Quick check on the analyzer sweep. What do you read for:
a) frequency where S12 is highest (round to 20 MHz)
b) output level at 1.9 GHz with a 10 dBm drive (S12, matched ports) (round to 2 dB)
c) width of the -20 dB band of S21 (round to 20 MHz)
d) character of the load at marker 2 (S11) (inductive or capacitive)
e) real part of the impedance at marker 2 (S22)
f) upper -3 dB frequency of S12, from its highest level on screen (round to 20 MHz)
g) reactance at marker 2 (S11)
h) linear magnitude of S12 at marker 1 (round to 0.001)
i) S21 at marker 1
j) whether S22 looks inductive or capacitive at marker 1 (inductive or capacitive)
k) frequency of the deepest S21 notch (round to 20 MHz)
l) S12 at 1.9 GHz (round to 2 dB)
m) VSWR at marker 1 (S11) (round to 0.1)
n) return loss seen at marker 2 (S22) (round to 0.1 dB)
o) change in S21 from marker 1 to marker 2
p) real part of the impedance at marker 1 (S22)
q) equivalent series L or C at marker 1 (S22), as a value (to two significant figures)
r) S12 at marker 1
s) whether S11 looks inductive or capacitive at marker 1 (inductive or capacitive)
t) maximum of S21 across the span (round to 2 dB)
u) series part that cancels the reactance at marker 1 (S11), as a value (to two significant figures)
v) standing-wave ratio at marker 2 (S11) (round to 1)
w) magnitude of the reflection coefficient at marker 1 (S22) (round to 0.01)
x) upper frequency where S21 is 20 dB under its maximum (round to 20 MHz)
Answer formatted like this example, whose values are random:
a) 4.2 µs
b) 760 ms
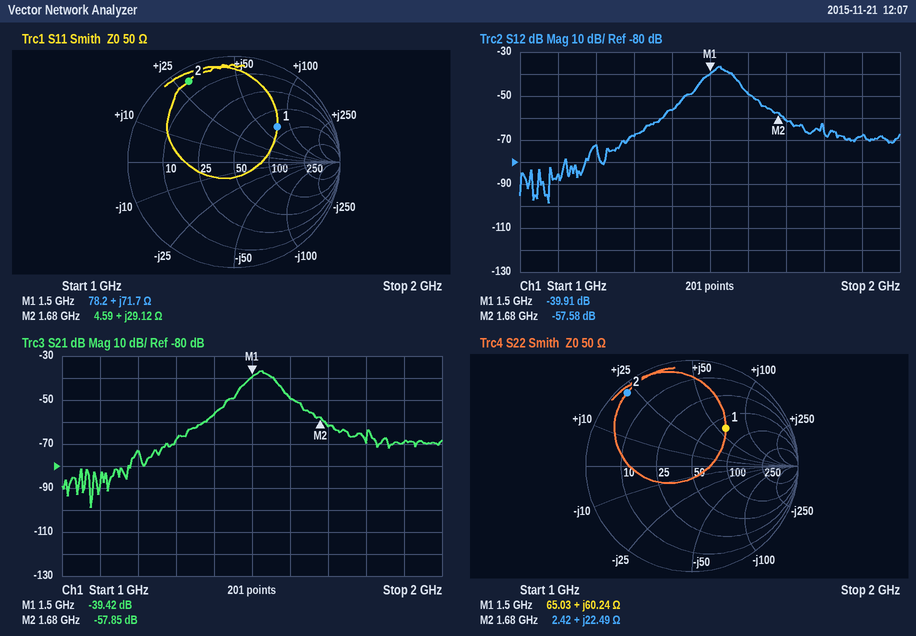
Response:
a) 1.52 GHz
b) -58 dBm
c) 260 MHz
d) inductive
e) 2.42 Ω
f) 1.56 GHz
g) +29.12 Ω
h) 0.010
i) -39.42 dB
j) inductive
k) 1.08 GHz
l) -68 dB
m) 3.2
n) 0.7 dB
o) -18.43 dB
p) 65.03 Ω
q) 6.4 nH
r) -39.91 dB
s) inductive
t) -36 dB
u) 1.5 pF
v) 15
w) 0.48
x) 1.66 GHz
